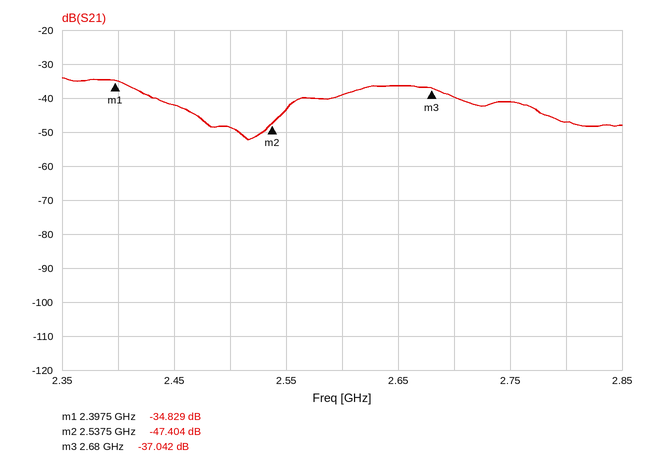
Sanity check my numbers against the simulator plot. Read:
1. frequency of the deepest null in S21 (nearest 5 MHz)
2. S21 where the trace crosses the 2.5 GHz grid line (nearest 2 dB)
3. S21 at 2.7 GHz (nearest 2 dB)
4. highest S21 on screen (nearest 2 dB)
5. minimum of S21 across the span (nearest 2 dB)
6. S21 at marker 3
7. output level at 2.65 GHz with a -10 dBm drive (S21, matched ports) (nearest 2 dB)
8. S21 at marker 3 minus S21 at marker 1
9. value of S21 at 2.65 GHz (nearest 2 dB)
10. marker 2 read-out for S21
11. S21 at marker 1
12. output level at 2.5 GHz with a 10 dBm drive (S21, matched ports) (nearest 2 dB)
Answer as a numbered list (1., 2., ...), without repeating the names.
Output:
1. 2.515 GHz
2. -48 dB
3. -40 dB
4. -34 dB
5. -52 dB
6. -37.042 dB
7. -46 dBm
8. -2.213 dB
9. -36 dB
10. -47.404 dB
11. -34.829 dB
12. -38 dBm
